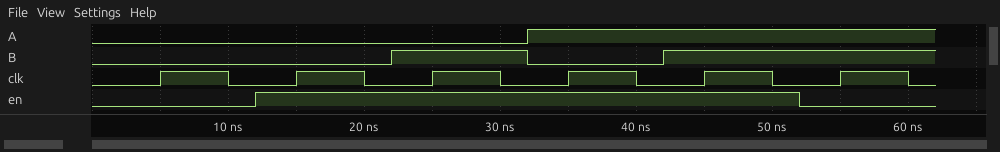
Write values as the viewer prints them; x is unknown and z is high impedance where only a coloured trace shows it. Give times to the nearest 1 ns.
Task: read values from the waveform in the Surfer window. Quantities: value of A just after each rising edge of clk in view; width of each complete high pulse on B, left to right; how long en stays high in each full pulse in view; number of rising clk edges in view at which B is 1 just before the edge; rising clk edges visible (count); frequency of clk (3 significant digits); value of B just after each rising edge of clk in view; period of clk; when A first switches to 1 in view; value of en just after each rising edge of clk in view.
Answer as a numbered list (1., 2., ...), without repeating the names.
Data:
1. 0 0 0 1 1 1
2. 10 ns
3. 40 ns
4. 3
5. 6
6. 100 MHz
7. 0 0 1 0 1 1
8. 10 ns
9. 32 ns
10. 0 1 1 1 1 0
